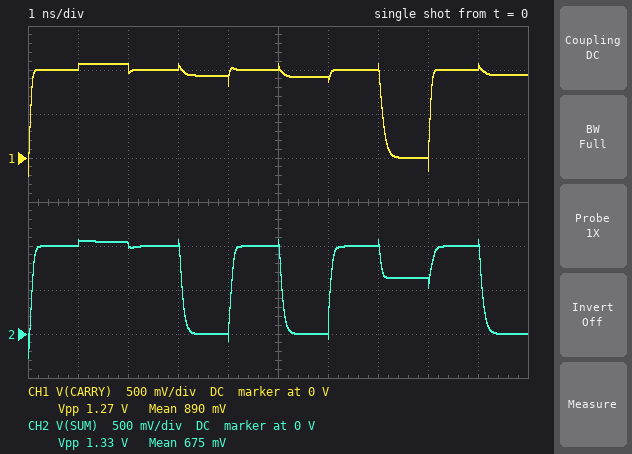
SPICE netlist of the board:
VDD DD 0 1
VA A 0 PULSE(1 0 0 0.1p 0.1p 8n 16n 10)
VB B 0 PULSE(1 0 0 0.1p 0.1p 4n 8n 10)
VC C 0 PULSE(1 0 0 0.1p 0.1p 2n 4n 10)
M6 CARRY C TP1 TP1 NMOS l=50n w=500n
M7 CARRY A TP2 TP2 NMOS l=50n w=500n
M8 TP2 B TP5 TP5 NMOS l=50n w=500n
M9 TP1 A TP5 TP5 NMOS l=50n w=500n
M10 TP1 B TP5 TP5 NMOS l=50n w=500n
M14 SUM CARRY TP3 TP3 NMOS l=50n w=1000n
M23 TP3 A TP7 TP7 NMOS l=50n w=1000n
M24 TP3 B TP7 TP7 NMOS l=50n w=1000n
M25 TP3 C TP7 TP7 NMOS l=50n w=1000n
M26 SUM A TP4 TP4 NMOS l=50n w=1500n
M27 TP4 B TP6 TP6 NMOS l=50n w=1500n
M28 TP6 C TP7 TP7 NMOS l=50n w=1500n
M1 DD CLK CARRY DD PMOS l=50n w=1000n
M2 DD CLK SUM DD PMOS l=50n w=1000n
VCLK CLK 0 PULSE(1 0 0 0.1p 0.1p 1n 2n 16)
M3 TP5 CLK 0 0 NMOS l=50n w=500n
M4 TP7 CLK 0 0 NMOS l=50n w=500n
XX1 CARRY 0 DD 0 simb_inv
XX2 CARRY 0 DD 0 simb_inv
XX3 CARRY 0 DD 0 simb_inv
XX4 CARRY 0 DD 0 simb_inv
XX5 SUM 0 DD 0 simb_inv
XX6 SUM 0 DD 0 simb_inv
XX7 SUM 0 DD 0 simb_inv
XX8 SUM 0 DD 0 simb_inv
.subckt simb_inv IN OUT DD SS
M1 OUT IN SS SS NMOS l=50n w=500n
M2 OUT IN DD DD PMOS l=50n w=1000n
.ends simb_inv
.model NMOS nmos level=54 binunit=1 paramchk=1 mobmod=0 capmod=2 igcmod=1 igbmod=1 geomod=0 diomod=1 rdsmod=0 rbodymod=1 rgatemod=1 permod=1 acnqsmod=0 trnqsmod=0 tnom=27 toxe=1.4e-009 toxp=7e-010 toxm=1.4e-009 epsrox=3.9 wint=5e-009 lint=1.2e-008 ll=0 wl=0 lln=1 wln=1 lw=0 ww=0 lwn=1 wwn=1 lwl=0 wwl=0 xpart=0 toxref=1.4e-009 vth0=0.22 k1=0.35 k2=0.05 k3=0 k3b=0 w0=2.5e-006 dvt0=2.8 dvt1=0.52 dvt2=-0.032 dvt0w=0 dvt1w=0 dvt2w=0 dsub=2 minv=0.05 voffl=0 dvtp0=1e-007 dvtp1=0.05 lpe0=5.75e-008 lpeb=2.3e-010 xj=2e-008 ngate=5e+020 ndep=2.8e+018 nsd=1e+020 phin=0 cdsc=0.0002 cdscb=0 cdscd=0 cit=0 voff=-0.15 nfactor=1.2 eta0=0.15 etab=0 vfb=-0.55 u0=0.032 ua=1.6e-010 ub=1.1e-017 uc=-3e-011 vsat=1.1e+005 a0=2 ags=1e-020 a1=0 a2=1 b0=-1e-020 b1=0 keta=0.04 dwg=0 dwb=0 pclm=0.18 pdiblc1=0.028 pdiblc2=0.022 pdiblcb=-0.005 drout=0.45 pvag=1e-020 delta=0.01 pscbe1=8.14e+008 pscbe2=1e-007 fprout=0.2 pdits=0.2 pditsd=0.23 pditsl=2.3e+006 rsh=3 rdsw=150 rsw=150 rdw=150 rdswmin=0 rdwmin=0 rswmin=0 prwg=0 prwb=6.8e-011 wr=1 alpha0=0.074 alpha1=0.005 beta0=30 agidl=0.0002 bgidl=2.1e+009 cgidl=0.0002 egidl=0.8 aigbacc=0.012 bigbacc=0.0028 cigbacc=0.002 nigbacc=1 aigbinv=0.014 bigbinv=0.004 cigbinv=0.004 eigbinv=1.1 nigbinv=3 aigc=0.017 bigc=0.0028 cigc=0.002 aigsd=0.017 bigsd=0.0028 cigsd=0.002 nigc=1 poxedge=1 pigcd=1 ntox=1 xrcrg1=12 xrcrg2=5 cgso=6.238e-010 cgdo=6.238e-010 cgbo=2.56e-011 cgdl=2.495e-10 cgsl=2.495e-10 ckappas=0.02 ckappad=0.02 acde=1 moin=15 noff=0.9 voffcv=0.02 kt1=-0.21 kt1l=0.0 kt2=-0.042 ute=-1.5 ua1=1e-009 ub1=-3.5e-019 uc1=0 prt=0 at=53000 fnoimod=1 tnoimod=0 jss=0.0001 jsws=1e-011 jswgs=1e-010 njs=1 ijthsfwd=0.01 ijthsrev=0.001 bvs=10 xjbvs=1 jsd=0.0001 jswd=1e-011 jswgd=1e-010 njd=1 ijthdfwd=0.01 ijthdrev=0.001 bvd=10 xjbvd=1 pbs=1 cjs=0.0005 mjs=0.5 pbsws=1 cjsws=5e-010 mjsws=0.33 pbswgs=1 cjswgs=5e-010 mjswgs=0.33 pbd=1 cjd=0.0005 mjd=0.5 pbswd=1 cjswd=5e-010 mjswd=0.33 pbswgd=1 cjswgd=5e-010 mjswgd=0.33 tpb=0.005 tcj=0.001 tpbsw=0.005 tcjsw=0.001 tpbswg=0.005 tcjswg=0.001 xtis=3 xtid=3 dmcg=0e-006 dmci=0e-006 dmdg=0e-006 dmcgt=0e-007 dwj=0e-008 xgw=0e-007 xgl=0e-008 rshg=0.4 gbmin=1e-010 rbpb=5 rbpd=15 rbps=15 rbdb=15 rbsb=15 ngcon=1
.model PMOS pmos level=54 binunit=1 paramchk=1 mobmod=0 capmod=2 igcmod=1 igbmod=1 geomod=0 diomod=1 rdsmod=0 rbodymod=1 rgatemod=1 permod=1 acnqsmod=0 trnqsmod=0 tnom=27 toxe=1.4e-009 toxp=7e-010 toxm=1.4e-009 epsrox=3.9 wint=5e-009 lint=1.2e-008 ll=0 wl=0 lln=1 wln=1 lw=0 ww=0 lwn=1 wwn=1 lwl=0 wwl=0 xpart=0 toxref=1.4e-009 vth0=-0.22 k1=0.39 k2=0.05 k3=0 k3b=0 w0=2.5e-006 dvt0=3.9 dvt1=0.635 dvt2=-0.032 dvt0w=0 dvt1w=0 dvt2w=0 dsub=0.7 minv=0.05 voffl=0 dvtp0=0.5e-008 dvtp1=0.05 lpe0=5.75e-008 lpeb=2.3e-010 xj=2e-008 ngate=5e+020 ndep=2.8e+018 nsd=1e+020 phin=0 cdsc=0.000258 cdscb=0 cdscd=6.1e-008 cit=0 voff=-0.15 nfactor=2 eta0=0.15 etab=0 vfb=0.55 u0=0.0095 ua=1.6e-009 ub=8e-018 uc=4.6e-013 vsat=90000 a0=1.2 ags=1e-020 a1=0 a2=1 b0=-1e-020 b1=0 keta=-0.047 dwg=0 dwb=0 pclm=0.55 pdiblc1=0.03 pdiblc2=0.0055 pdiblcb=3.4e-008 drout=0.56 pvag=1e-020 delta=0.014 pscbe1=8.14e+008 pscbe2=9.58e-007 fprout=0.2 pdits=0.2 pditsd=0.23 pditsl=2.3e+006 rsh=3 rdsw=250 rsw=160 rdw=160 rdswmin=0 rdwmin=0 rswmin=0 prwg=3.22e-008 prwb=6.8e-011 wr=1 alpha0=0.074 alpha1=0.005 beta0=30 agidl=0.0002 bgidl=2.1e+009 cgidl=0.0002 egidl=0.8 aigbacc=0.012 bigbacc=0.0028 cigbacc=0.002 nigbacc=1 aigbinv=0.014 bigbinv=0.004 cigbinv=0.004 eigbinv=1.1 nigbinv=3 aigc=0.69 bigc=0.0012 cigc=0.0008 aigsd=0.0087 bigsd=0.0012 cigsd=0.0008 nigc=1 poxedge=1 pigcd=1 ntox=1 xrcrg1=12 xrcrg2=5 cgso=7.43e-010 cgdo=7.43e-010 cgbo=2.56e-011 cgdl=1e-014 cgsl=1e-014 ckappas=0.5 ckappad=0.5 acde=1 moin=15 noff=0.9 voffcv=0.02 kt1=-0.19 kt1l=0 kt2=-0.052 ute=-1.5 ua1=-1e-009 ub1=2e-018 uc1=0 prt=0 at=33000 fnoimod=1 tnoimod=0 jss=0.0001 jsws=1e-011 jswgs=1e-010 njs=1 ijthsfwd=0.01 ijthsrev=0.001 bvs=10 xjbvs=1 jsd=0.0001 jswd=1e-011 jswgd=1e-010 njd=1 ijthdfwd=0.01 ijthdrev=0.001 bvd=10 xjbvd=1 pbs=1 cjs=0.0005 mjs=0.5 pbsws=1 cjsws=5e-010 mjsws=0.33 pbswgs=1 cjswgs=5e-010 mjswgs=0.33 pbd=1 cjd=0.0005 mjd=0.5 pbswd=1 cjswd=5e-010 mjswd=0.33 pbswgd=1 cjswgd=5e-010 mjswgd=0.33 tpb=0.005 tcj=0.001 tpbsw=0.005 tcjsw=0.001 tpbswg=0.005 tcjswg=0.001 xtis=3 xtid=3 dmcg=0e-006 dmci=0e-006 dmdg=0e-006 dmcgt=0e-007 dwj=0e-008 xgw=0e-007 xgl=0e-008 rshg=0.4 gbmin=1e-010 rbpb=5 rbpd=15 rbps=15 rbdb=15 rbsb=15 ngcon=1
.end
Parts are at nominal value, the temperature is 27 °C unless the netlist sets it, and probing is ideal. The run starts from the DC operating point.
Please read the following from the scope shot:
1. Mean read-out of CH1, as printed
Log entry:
890 mV
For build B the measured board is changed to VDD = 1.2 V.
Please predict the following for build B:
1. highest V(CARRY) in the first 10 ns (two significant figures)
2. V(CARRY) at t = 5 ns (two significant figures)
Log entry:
1.3 V
1.2 V
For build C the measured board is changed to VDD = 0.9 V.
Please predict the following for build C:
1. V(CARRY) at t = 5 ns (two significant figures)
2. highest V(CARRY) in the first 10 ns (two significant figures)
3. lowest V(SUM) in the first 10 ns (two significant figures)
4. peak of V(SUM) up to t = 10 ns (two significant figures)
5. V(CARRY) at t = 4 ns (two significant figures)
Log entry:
900 mV
970 mV
-280 mV
960 mV
850 mV
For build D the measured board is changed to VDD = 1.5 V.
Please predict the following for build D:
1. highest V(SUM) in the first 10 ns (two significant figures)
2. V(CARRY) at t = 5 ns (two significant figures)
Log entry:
1.6 V
1.5 V
